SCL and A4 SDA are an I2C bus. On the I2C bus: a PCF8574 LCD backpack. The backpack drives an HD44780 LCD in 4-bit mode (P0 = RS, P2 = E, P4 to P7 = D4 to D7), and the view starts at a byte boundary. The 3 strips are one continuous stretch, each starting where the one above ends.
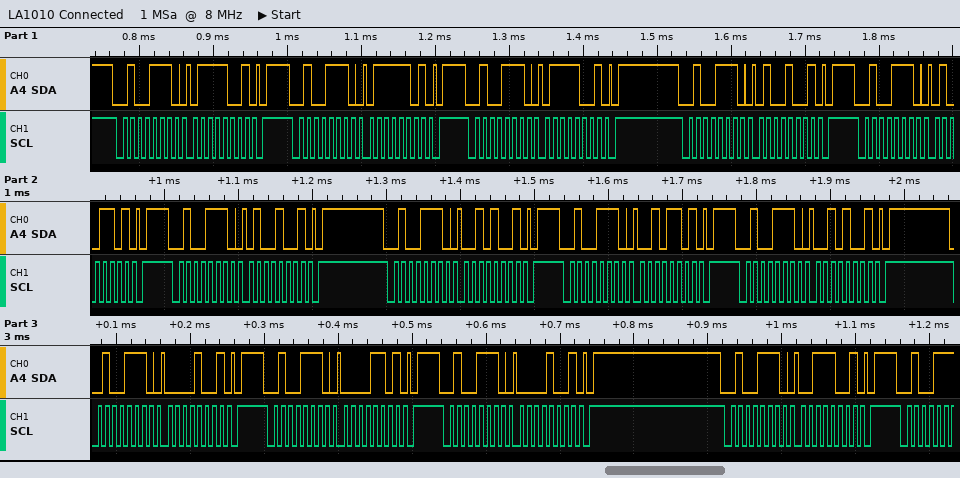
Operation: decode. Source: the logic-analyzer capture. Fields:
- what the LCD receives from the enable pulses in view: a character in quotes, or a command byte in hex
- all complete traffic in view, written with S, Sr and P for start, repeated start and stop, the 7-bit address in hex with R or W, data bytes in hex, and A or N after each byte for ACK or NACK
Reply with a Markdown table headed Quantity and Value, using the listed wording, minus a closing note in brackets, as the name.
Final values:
| Quantity | Value |
|---|---|
| what the LCD receives from the enable pulses in view: a character in quotes, or a command byte in hex | 't' ' ' |
| all complete traffic in view, written with S, Sr and P for start, repeated start and stop, the 7-bit address in hex with R or W, data bytes in hex, and A or N after each byte for ACK or NACK | S 27W A 79 A P S 27W A 7D A P S 27W A 79 A P S 27W A 49 A P S 27W A 4D A P S 27W A 49 A P S 27W A 29 A P S 27W A 2D A P S 27W A 29 A P S 27W A 09 A P S 27W A 0D A P S 27W A 09 A P S 27W A 39 A P |
